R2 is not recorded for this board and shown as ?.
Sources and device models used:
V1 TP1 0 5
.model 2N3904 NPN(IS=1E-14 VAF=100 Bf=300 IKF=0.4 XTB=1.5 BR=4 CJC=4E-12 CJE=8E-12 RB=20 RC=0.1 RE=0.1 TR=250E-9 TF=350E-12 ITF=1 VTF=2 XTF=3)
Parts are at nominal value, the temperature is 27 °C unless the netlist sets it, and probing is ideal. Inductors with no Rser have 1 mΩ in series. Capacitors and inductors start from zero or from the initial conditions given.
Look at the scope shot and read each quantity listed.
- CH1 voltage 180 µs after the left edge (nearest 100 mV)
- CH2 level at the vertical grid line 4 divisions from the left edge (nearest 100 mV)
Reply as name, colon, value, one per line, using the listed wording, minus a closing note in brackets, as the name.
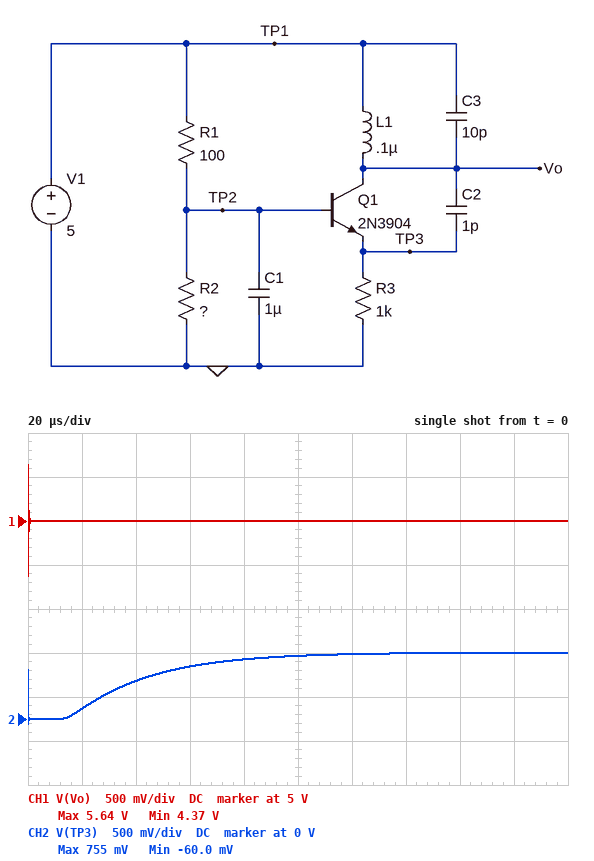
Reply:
CH1 voltage 180 µs after the left edge: 5.0 V
CH2 level at the vertical grid line 4 divisions from the left edge: 700 mV
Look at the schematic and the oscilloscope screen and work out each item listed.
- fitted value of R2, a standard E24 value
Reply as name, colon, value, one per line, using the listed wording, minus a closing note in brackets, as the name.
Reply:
fitted value of R2, a standard E24 value: 39 Ω
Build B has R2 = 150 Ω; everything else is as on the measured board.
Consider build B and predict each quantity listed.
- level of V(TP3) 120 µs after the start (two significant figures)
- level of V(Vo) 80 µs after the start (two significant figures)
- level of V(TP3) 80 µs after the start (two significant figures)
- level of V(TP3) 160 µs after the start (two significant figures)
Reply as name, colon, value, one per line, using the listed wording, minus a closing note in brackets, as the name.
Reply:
level of V(TP3) 120 µs after the start: 1.9 V
level of V(Vo) 80 µs after the start: 5.0 V
level of V(TP3) 80 µs after the start: 1.5 V
level of V(TP3) 160 µs after the start: 2.1 V
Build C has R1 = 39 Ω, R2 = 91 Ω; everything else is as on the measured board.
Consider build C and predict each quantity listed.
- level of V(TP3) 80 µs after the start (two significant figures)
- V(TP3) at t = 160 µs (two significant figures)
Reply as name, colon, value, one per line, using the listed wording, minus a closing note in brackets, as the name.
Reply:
level of V(TP3) 80 µs after the start: 2.6 V
V(TP3) at t = 160 µs: 2.8 V
